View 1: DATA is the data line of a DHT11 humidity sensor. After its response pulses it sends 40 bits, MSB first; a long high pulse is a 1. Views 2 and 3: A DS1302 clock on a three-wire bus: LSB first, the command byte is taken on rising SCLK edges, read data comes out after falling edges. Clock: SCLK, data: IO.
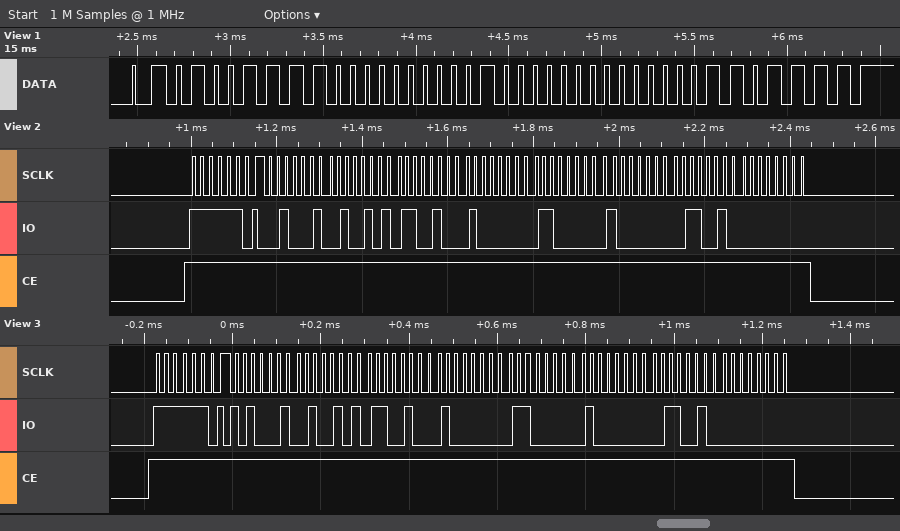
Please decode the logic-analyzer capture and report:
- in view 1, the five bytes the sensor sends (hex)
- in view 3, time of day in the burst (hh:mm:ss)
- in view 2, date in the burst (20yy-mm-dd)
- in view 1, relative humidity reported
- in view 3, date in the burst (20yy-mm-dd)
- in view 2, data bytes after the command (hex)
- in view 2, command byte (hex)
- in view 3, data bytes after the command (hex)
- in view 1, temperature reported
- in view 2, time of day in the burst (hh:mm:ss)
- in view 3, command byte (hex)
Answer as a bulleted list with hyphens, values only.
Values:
- 4F 00 20 00 6F
- 13:52:45
- 2026-03-01
- 79 %
- 2026-03-01
- 44 52 13 01 03 01 26 00
- 0xBF
- 45 52 13 01 03 01 26 00
- 32.0 °C
- 13:52:44
- 0xBF
